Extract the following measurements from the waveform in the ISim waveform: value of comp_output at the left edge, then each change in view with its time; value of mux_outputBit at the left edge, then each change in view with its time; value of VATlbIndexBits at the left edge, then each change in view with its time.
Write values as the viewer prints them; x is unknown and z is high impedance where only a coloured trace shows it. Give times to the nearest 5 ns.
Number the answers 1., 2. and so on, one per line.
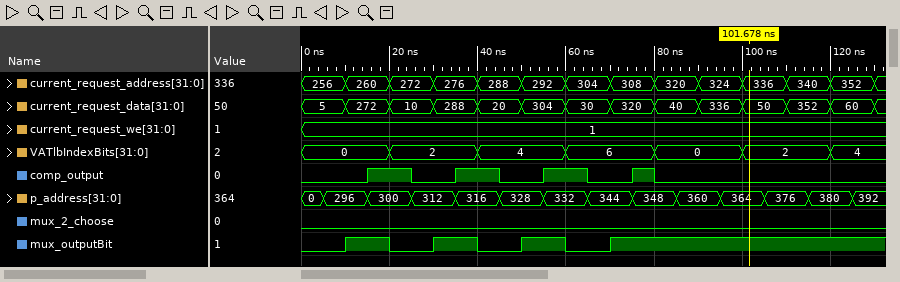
1. 0, 1 at 15 ns, 0 at 25 ns, 1 at 35 ns, 0 at 45 ns, 1 at 55 ns, 0 at 65 ns, 1 at 75 ns, 0 at 80 ns
2. 0, 1 at 10 ns, 0 at 20 ns, 1 at 30 ns, 0 at 40 ns, 1 at 50 ns, 0 at 60 ns, 1 at 70 ns
3. 0, 2 at 20 ns, 4 at 40 ns, 6 at 60 ns, 0 at 80 ns, 2 at 100 ns, 4 at 120 ns
